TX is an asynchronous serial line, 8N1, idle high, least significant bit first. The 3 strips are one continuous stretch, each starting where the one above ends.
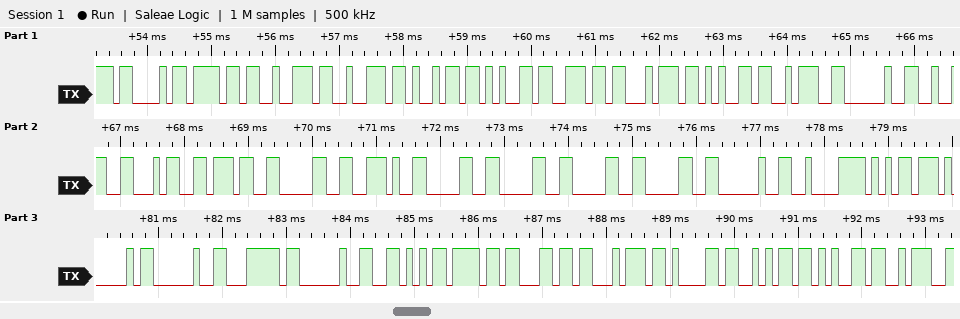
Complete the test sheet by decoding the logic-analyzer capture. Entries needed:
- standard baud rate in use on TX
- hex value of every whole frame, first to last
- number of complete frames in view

9600 baud
0x43 0x6F 0x72 0x72 0x69 0x65 0x6E 0x74 0x65 0x3A 0x20 0x32 0x34 0x37 0x30 0x2E 0x30 0x30 0x30 0x30 0x20 0xC2 0xB5 0x41 0x20 0x7C 0x20 0x56 0x6F 0x6C 0x74 0x61 0x6A 0x65 0x3A
35
